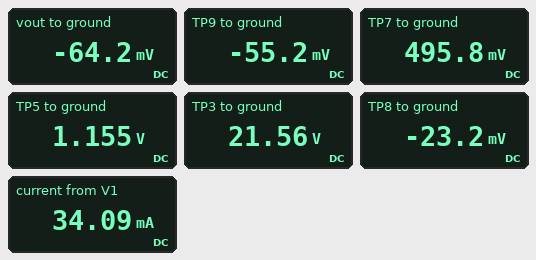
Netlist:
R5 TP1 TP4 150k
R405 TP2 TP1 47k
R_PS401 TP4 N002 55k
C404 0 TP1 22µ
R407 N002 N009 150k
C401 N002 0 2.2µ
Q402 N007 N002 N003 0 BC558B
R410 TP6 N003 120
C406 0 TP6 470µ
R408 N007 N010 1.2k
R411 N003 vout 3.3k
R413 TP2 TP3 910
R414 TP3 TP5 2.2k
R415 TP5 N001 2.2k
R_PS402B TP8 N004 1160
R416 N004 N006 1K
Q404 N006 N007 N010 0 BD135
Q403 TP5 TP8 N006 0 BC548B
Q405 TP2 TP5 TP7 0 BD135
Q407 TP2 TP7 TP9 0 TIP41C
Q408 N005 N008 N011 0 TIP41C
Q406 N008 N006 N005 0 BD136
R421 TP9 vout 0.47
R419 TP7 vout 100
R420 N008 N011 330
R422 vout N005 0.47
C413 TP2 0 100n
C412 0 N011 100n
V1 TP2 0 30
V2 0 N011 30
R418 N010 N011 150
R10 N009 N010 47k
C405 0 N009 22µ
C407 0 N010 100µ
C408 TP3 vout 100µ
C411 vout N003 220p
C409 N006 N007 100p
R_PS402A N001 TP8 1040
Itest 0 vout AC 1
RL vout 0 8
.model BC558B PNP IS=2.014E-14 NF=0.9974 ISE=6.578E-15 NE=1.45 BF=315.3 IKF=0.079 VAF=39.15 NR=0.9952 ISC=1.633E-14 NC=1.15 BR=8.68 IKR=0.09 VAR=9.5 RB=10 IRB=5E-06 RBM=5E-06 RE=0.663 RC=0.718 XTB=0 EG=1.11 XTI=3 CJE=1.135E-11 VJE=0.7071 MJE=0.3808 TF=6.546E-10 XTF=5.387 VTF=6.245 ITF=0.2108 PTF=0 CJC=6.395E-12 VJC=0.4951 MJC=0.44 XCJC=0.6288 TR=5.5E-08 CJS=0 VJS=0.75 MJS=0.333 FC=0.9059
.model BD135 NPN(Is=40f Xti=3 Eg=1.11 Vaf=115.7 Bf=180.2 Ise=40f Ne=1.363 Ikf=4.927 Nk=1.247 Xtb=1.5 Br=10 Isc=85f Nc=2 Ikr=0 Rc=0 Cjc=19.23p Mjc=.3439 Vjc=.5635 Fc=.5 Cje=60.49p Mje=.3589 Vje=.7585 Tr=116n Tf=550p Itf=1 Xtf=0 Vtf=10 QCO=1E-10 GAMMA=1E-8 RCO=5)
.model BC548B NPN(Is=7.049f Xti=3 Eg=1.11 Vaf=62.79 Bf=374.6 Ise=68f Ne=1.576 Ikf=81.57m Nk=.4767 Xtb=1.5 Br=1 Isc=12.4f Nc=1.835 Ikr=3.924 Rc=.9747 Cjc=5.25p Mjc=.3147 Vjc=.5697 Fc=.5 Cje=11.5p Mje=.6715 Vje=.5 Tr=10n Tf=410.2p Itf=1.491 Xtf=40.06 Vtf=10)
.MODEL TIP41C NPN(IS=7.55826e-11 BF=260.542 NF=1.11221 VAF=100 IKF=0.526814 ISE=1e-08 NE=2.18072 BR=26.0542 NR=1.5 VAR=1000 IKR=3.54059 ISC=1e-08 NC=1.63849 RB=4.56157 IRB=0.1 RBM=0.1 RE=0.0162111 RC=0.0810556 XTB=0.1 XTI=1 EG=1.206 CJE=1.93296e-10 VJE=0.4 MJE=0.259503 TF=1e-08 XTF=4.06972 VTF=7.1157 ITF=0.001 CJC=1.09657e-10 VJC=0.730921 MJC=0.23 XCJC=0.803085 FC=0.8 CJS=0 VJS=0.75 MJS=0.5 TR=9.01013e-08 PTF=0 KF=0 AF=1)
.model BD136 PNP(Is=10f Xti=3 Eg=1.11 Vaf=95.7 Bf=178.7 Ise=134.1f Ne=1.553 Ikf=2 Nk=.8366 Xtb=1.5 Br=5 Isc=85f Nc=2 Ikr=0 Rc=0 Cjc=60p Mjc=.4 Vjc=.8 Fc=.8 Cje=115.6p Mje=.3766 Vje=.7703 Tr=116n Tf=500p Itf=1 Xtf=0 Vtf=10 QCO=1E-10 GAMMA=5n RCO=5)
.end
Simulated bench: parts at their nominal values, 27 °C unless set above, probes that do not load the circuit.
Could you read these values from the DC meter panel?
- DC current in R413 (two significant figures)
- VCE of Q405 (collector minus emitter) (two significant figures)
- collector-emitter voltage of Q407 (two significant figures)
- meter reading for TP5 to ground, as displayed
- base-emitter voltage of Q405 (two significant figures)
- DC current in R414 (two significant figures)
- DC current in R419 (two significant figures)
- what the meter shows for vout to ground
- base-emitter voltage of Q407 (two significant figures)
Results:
9.3 mA
30 V
30 V
1.155 V
660 mV
9.3 mA
5.6 mA
-64.2 mV
550 mV
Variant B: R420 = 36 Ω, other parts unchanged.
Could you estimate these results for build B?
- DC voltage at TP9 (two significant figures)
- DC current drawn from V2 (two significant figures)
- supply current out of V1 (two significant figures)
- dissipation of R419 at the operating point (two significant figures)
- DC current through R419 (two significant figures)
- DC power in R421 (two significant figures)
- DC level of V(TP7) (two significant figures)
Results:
-53 mV
28 mA
21 mA
2.7 mW
5.2 mA
17 µW
460 mV
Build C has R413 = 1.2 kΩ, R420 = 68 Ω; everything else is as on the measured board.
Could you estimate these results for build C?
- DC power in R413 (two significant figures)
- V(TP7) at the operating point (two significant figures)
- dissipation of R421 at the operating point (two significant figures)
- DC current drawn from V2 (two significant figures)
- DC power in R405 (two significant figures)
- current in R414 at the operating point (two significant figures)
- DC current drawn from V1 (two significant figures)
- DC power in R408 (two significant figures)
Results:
87 mW
370 mV
12 µW
37 mA
790 µW
8.5 mA
19 mA
370 µW
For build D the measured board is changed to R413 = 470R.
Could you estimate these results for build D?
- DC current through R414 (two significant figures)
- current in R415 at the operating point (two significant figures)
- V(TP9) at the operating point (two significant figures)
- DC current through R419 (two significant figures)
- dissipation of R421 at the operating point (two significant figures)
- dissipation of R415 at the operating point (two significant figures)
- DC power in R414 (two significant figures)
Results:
11 mA
370 µA
110 mV
5.9 mA
600 µW
300 µW
250 mW
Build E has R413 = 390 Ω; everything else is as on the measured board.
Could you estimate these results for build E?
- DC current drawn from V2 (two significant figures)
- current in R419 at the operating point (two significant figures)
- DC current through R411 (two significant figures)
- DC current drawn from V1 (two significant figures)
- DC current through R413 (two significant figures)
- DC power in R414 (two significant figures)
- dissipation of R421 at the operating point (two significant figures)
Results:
40 mA
5.9 mA
620 µA
57 mA
11 mA
270 mW
740 µW
